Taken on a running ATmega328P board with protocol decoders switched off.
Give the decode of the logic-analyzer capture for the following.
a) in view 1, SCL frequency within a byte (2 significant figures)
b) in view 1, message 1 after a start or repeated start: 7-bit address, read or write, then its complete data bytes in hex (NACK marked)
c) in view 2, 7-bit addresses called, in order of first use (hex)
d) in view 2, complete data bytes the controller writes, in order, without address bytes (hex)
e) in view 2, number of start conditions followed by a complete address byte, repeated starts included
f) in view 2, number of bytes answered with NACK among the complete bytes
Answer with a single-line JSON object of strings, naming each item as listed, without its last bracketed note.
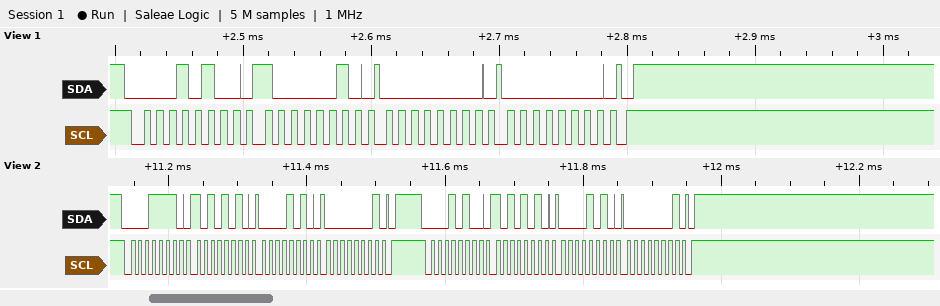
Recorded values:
{"in view 1, SCL frequency within a byte": "100 kHz", "in view 1, message 1 after a start or repeated start: 7-bit address, read or write, then its complete data bytes in hex": "0x0A write: 82 00 00", "in view 2, 7-bit addresses called, in order of first use": "0x0F 0x0A", "in view 2, complete data bytes the controller writes, in order, without address bytes": "AA 0A 01 AA 0A 01", "in view 2, number of start conditions followed by a complete address byte, repeated starts included": "2", "in view 2, number of bytes answered with NACK among the complete bytes": "0"}
